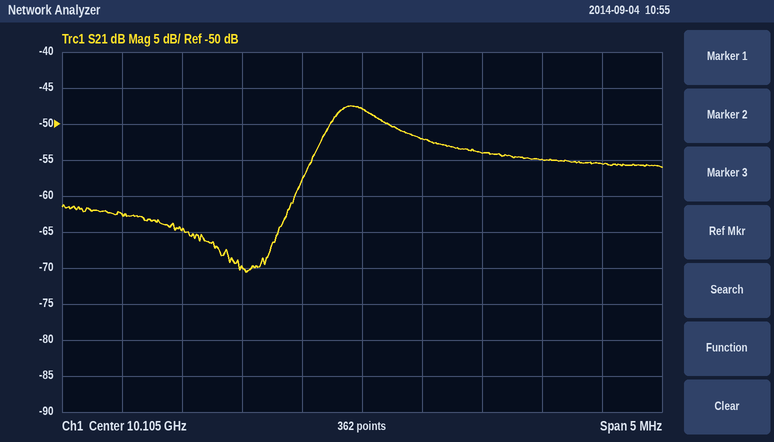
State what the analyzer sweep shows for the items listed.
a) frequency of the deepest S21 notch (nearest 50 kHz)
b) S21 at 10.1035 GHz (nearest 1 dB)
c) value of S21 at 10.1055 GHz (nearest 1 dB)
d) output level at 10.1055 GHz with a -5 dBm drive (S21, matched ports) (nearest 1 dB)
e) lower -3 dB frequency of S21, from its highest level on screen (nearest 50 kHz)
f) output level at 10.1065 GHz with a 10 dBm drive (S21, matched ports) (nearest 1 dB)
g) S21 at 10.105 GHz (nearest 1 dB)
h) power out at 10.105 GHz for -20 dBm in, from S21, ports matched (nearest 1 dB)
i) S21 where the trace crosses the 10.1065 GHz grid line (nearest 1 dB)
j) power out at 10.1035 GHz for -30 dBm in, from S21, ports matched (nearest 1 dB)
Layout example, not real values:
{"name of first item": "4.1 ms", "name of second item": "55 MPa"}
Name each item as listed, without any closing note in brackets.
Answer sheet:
{"frequency of the deepest S21 notch": "10.10405 GHz", "S21 at 10.1035 GHz": "-65 dB", "value of S21 at 10.1055 GHz": "-52 dB", "output level at 10.1055 GHz with a -5 dBm drive (S21, matched ports)": "-57 dBm", "lower -3 dB frequency of S21, from its highest level on screen": "10.10470 GHz", "output level at 10.1065 GHz with a 10 dBm drive (S21, matched ports)": "-45 dBm", "S21 at 10.105 GHz": "-48 dB", "power out at 10.105 GHz for -20 dBm in, from S21, ports matched": "-68 dBm", "S21 where the trace crosses the 10.1065 GHz grid line": "-55 dB", "power out at 10.1035 GHz for -30 dBm in, from S21, ports matched": "-95 dBm"}
